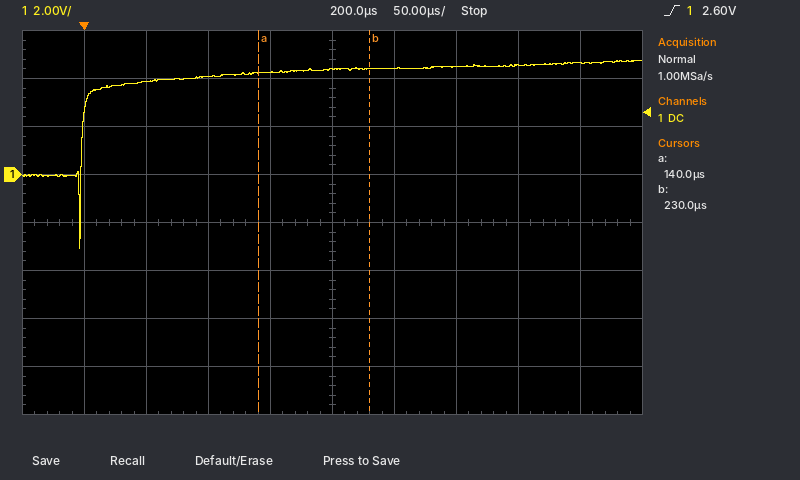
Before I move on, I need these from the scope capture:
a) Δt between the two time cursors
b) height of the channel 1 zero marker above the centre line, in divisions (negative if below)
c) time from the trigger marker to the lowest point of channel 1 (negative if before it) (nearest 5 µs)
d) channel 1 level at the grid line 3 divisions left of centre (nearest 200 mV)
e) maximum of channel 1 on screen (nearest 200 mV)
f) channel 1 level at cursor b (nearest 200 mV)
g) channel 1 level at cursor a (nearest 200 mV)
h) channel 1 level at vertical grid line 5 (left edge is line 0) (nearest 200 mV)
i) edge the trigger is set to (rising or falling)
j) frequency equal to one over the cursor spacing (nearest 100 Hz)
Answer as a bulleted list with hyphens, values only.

- 90 µs
- +1.0 div
- -5 µs
- 3.8 V
- 4.8 V
- 4.4 V
- 4.2 V
- 4.4 V
- rising
- 11.1 kHz
